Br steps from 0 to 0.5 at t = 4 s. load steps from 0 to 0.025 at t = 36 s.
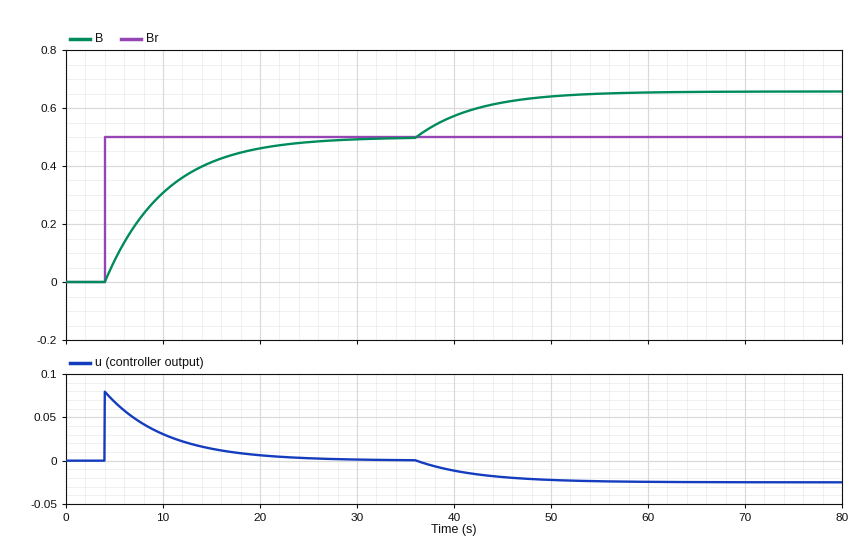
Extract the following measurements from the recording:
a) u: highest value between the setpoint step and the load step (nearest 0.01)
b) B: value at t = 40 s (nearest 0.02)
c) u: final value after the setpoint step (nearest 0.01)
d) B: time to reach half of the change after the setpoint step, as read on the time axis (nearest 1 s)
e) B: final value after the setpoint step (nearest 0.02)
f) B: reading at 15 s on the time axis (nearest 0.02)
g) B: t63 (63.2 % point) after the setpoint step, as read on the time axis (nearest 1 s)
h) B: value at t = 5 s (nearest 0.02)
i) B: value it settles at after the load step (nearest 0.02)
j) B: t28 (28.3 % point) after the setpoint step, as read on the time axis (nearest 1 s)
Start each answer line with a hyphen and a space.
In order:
- 0.08
- 0.58
- 0.00
- 8 s
- 0.50
- 0.42
- 10 s
- 0.08
- 0.66
- 6 s
